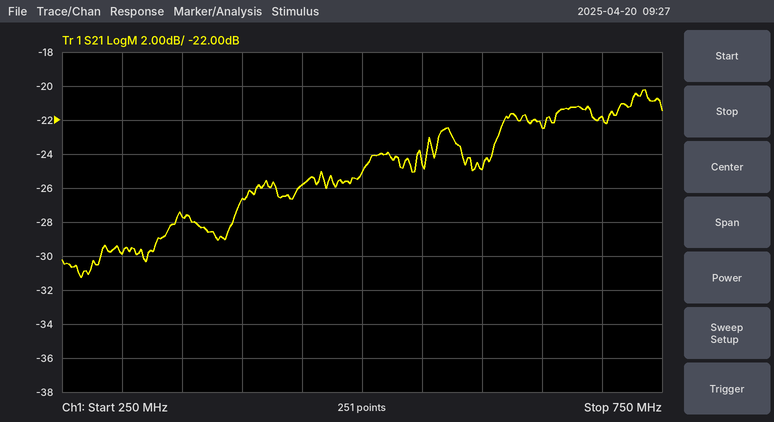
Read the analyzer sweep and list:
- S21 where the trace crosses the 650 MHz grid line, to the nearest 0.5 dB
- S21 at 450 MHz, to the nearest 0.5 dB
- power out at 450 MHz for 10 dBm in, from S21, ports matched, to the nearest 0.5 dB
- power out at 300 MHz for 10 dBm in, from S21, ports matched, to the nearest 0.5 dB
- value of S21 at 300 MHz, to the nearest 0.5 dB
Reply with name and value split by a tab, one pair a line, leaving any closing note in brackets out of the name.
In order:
S21 where the trace crosses the 650 MHz grid line, to the nearest 0.5 dB	-22.5 dB
S21 at 450 MHz, to the nearest 0.5 dB	-26.0 dB
power out at 450 MHz for 10 dBm in, from S21, ports matched, to the nearest 0.5 dB	-16.0 dBm
power out at 300 MHz for 10 dBm in, from S21, ports matched, to the nearest 0.5 dB	-20.0 dBm
value of S21 at 300 MHz, to the nearest 0.5 dB	-30.0 dB
